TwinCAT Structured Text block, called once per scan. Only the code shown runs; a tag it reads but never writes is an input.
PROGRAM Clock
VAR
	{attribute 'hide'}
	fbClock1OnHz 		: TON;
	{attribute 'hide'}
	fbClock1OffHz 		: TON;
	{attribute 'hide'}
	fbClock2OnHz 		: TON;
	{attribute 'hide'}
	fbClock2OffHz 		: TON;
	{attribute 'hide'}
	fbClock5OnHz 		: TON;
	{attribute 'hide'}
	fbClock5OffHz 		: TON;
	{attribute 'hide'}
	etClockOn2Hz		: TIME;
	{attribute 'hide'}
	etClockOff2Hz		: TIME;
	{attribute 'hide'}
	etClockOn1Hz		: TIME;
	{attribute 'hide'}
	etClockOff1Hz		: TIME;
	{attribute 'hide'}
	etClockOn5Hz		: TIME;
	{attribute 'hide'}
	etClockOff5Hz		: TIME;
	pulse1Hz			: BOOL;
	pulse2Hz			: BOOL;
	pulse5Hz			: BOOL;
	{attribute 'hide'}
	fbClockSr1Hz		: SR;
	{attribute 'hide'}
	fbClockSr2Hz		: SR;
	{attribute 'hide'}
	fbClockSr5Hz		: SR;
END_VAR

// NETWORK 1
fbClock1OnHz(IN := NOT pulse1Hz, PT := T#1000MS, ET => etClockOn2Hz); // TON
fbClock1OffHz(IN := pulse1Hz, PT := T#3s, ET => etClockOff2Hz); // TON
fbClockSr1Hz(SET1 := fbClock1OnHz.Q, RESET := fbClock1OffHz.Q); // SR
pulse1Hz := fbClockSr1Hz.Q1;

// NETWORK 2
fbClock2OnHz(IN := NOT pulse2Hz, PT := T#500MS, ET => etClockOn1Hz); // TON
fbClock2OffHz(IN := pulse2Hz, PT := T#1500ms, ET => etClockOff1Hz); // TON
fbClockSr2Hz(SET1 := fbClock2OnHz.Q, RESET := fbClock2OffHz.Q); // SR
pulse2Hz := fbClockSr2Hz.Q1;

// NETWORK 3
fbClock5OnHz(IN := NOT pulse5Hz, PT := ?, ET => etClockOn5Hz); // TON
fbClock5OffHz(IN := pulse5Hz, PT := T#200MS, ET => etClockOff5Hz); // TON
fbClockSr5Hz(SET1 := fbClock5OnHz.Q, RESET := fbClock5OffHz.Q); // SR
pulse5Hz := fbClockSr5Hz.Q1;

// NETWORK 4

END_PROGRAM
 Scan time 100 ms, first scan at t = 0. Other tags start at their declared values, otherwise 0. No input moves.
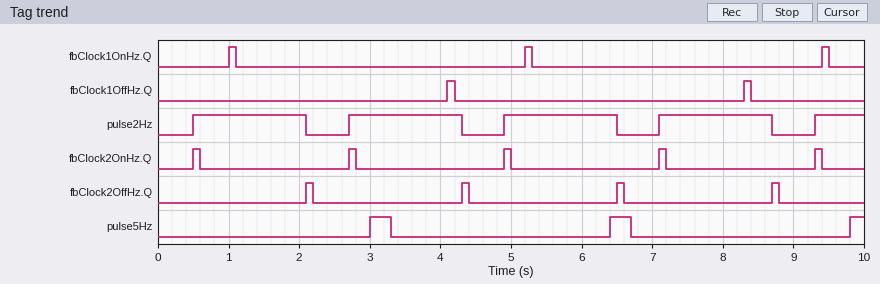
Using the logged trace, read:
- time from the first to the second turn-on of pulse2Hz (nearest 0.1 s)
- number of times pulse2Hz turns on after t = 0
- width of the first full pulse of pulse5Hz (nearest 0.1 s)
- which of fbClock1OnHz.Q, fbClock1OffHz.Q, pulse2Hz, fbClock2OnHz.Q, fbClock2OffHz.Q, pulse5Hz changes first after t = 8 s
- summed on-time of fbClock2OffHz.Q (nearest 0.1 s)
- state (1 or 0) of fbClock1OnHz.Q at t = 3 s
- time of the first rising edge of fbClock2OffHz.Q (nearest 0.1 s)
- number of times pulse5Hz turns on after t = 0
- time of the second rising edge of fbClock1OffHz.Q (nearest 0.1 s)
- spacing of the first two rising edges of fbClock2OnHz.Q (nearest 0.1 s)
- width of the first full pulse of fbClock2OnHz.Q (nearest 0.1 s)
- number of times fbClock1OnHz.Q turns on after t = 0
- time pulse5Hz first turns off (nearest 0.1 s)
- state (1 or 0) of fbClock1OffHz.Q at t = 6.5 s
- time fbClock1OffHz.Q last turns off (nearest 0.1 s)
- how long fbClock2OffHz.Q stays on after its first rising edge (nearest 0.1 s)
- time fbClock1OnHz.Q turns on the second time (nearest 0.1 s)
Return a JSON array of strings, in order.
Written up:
["2.2 s", "5", "0.3 s", "fbClock1OffHz.Q", "0.4 s", "0", "2.1 s", "3", "8.3 s", "2.2 s", "0.1 s", "3", "3.3 s", "0", "8.4 s", "0.1 s", "5.2 s"]
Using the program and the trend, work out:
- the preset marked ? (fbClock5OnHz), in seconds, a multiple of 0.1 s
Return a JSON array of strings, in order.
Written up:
["3.0 s"]
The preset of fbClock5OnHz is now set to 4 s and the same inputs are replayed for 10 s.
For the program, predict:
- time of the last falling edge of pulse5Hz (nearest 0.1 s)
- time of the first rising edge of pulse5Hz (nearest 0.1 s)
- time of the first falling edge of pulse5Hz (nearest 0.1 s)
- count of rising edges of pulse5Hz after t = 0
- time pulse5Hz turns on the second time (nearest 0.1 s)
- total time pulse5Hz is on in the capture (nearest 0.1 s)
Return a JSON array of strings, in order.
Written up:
["8.7 s", "4.0 s", "4.3 s", "2", "8.4 s", "0.6 s"]
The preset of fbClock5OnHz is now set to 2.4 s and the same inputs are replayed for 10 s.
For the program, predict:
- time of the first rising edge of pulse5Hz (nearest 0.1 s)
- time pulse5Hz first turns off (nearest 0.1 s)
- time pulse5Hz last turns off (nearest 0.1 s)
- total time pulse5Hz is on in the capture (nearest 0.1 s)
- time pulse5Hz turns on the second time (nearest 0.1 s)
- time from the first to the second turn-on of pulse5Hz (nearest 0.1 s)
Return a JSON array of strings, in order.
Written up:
["2.4 s", "2.7 s", "8.3 s", "0.9 s", "5.2 s", "2.8 s"]
